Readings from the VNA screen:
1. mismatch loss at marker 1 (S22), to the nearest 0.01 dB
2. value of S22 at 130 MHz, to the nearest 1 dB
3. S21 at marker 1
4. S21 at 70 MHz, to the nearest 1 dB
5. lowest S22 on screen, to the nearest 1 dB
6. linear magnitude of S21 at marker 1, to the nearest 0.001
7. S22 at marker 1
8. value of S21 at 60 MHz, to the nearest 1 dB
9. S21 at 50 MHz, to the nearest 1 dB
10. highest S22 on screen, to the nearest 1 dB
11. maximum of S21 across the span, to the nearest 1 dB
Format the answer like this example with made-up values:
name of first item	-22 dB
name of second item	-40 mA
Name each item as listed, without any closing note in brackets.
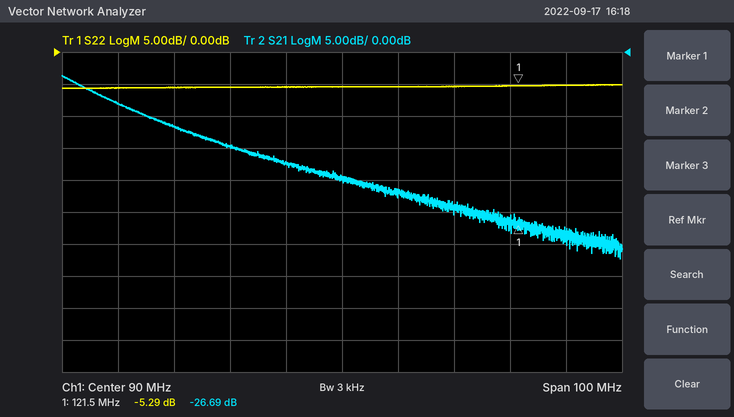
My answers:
mismatch loss at marker 1 (S22), to the nearest 0.01 dB	1.52 dB
value of S22 at 130 MHz, to the nearest 1 dB	-5 dB
S21 at marker 1	-26.69 dB
S21 at 70 MHz, to the nearest 1 dB	-15 dB
lowest S22 on screen, to the nearest 1 dB	-6 dB
linear magnitude of S21 at marker 1, to the nearest 0.001	0.046
S22 at marker 1	-5.29 dB
value of S21 at 60 MHz, to the nearest 1 dB	-12 dB
S21 at 50 MHz, to the nearest 1 dB	-8 dB
highest S22 on screen, to the nearest 1 dB	-5 dB
maximum of S21 across the span, to the nearest 1 dB	-4 dB
